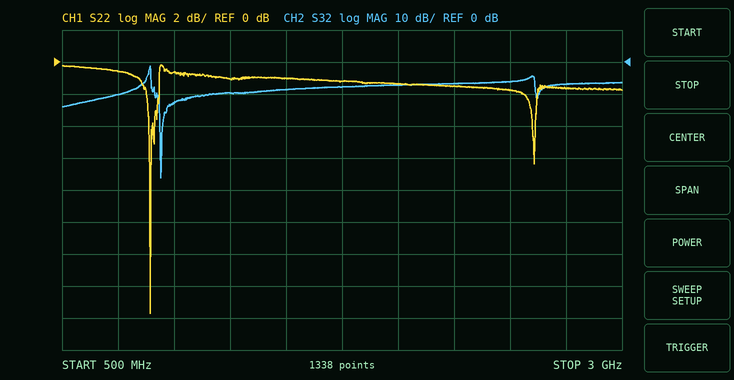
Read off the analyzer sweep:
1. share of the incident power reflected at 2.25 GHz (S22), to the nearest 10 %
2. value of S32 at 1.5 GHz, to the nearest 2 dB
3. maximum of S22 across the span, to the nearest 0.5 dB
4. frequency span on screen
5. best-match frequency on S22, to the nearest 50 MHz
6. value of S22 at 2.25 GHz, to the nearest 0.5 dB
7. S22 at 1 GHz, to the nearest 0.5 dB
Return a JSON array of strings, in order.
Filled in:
["70 %", "-8 dB", "0.0 dB", "2.5 GHz", "900 MHz", "-1.5 dB", "-0.5 dB"]
